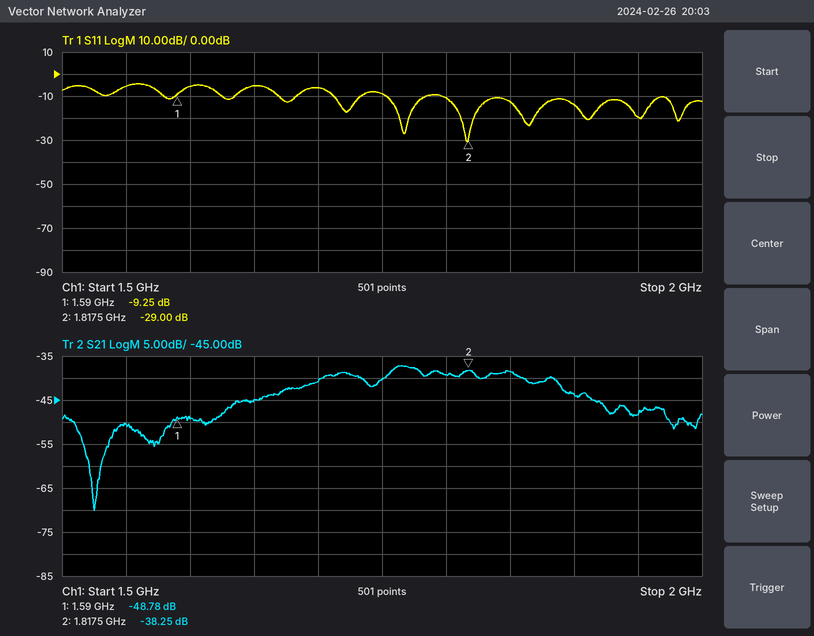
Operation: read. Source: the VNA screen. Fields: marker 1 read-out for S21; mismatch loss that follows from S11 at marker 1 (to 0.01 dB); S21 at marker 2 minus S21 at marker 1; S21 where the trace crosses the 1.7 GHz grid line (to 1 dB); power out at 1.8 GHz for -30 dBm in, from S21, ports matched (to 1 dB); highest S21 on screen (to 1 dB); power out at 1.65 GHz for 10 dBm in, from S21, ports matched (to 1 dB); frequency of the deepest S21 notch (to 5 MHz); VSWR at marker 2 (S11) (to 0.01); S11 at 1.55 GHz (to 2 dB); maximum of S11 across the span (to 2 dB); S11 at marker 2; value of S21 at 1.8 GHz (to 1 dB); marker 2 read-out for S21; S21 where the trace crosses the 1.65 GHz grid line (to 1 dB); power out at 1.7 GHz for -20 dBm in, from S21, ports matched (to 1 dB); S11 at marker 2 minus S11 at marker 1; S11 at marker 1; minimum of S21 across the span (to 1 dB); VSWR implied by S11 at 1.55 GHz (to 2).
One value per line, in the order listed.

-48.78 dB
0.55 dB
10.53 dB
-41 dB
-69 dBm
-37 dB
-35 dBm
1.525 GHz
1.07
-6 dB
-4 dB
-29.00 dB
-39 dB
-38.25 dB
-45 dB
-61 dBm
-19.75 dB
-9.25 dB
-70 dB
4
